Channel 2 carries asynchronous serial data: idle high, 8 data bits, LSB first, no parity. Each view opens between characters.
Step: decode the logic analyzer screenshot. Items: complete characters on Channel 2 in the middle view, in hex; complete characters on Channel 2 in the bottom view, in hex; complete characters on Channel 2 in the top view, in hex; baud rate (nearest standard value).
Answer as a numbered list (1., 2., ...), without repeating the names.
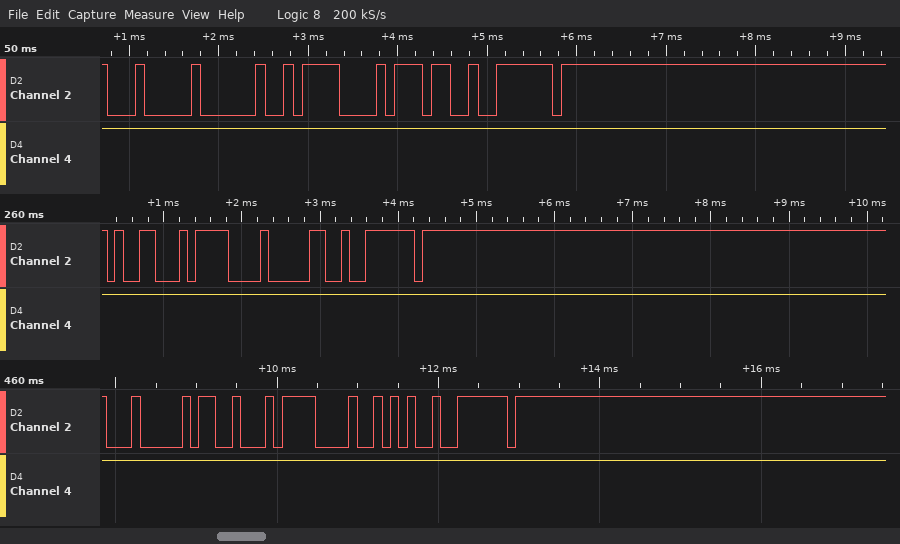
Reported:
1. 19, 0F, 30, 7E
2. 04, 13, 0F, 2A, 7E
3. 04, 20, 0F, 37, 7E
4. 9600 baud
